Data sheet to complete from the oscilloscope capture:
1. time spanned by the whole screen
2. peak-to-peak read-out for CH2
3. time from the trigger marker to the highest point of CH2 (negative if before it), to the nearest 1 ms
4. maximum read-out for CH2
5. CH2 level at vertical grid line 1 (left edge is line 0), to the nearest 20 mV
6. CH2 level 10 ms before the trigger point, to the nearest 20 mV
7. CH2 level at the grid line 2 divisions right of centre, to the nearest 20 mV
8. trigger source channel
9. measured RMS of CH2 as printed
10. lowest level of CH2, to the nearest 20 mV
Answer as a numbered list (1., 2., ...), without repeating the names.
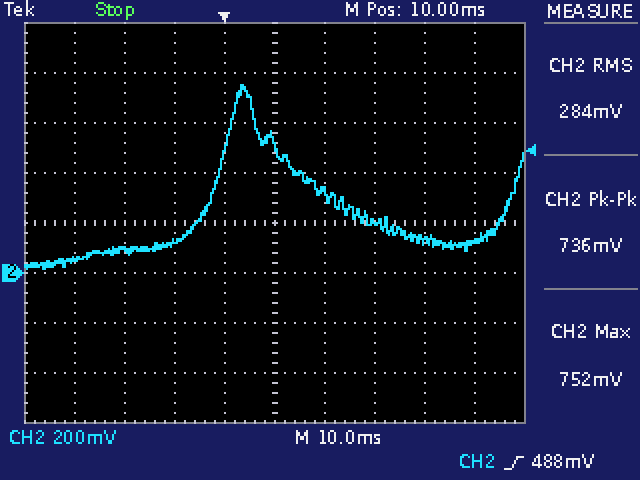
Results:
1. 100 ms
2. 736 mV
3. +4 ms
4. 752 mV
5. 60 mV
6. 120 mV
7. 200 mV
8. CH2
9. 284 mV
10. 20 mV
